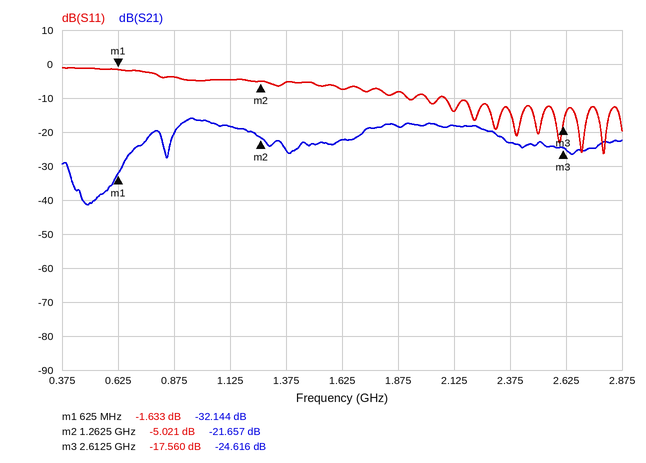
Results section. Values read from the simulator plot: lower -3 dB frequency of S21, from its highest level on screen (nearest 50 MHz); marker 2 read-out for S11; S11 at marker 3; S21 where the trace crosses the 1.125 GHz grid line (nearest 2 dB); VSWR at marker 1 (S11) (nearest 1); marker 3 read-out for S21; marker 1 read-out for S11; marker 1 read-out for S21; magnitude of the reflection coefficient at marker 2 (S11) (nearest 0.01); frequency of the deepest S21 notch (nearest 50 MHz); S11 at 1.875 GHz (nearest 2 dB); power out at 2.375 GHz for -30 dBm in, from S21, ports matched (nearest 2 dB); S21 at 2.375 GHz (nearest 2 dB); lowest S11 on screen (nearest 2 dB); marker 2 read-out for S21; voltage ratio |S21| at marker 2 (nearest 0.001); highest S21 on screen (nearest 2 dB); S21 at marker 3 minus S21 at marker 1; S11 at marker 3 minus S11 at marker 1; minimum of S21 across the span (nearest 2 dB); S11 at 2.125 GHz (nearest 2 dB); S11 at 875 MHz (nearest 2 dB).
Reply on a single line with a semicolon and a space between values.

900 MHz; -5.021 dB; -17.560 dB; -18 dB; 11; -24.616 dB; -1.633 dB; -32.144 dB; 0.56; 500 MHz; -8 dB; -54 dBm; -24 dB; -26 dB; -21.657 dB; 0.083; -16 dB; 7.528 dB; -15.927 dB; -42 dB; -14 dB; -4 dB
